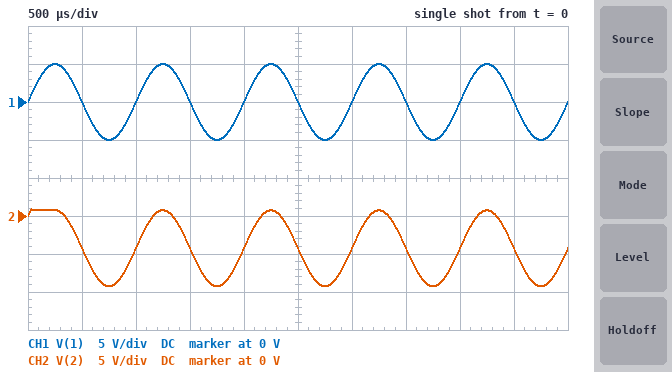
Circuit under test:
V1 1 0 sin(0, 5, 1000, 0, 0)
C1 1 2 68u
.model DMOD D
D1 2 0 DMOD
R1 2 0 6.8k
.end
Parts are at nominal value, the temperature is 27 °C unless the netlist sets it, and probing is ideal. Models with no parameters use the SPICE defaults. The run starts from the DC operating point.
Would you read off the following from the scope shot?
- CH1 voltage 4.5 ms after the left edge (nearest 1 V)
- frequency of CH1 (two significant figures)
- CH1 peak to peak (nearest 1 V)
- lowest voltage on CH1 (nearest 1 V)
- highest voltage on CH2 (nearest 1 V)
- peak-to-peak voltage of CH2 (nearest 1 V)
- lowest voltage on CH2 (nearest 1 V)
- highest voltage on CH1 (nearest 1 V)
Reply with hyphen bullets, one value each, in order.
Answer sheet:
- 0 V
- 1.0 kHz
- 10 V
- -5 V
- 1 V
- 10 V
- -9 V
- 5 V
